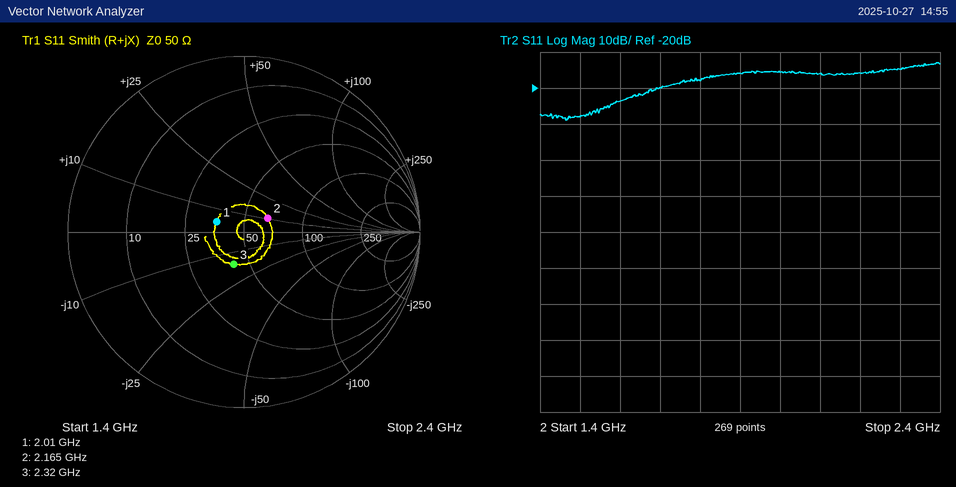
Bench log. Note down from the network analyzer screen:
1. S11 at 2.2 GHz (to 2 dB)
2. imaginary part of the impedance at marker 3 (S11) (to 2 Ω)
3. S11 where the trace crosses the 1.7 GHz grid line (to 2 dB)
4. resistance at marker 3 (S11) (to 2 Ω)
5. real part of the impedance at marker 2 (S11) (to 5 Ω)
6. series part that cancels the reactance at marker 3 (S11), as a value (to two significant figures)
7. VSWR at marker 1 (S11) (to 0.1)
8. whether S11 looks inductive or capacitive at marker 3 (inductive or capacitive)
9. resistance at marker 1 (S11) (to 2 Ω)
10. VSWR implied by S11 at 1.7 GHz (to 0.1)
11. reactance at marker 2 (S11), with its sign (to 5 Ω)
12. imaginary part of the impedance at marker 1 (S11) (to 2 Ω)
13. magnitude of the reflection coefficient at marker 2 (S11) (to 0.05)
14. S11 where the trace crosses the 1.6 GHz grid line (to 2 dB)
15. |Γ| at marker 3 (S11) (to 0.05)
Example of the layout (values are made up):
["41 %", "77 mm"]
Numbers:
["-16 dB", "-16 Ω", "-20 dB", "42 Ω", "65 Ω", "1.1 nH", "1.4", "capacitive", "36 Ω", "1.2", "+10 Ω", "+4 Ω", "0.15", "-24 dB", "0.20"]
